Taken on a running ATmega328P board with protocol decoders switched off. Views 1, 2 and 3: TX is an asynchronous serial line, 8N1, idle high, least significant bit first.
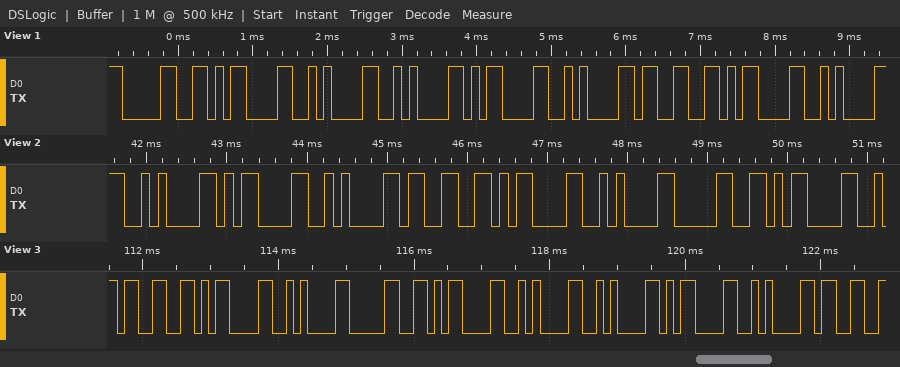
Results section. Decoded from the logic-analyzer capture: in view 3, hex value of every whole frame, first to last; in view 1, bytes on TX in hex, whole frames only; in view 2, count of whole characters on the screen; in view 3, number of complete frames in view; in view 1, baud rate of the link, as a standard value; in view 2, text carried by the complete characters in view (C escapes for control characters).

33 0D 0A 30 0D 0A 0A 0D 0A 33
30 0D 0A 0A 0D 0A 33 0D 0A
8
10
9600 baud
"\n\r\n3\r\n0\r"
